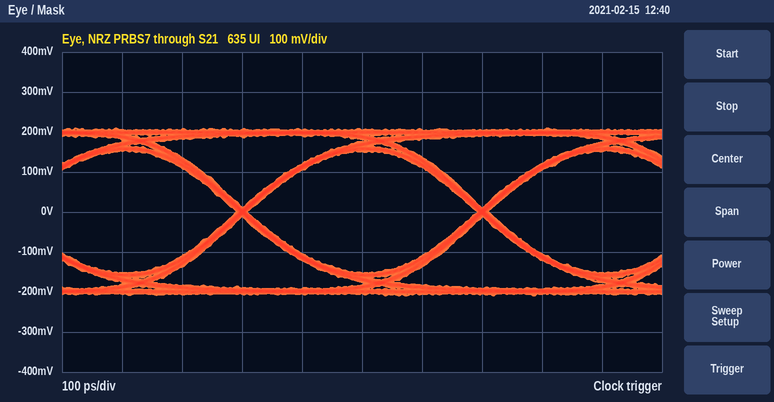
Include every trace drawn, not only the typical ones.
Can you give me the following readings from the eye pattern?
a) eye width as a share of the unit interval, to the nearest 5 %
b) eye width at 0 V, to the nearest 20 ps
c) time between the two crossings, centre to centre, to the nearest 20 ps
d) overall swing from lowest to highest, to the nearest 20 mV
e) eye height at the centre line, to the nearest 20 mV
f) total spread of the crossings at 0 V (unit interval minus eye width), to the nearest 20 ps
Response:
95 %
380 ps
400 ps
420 mV
300 mV
20 ps
